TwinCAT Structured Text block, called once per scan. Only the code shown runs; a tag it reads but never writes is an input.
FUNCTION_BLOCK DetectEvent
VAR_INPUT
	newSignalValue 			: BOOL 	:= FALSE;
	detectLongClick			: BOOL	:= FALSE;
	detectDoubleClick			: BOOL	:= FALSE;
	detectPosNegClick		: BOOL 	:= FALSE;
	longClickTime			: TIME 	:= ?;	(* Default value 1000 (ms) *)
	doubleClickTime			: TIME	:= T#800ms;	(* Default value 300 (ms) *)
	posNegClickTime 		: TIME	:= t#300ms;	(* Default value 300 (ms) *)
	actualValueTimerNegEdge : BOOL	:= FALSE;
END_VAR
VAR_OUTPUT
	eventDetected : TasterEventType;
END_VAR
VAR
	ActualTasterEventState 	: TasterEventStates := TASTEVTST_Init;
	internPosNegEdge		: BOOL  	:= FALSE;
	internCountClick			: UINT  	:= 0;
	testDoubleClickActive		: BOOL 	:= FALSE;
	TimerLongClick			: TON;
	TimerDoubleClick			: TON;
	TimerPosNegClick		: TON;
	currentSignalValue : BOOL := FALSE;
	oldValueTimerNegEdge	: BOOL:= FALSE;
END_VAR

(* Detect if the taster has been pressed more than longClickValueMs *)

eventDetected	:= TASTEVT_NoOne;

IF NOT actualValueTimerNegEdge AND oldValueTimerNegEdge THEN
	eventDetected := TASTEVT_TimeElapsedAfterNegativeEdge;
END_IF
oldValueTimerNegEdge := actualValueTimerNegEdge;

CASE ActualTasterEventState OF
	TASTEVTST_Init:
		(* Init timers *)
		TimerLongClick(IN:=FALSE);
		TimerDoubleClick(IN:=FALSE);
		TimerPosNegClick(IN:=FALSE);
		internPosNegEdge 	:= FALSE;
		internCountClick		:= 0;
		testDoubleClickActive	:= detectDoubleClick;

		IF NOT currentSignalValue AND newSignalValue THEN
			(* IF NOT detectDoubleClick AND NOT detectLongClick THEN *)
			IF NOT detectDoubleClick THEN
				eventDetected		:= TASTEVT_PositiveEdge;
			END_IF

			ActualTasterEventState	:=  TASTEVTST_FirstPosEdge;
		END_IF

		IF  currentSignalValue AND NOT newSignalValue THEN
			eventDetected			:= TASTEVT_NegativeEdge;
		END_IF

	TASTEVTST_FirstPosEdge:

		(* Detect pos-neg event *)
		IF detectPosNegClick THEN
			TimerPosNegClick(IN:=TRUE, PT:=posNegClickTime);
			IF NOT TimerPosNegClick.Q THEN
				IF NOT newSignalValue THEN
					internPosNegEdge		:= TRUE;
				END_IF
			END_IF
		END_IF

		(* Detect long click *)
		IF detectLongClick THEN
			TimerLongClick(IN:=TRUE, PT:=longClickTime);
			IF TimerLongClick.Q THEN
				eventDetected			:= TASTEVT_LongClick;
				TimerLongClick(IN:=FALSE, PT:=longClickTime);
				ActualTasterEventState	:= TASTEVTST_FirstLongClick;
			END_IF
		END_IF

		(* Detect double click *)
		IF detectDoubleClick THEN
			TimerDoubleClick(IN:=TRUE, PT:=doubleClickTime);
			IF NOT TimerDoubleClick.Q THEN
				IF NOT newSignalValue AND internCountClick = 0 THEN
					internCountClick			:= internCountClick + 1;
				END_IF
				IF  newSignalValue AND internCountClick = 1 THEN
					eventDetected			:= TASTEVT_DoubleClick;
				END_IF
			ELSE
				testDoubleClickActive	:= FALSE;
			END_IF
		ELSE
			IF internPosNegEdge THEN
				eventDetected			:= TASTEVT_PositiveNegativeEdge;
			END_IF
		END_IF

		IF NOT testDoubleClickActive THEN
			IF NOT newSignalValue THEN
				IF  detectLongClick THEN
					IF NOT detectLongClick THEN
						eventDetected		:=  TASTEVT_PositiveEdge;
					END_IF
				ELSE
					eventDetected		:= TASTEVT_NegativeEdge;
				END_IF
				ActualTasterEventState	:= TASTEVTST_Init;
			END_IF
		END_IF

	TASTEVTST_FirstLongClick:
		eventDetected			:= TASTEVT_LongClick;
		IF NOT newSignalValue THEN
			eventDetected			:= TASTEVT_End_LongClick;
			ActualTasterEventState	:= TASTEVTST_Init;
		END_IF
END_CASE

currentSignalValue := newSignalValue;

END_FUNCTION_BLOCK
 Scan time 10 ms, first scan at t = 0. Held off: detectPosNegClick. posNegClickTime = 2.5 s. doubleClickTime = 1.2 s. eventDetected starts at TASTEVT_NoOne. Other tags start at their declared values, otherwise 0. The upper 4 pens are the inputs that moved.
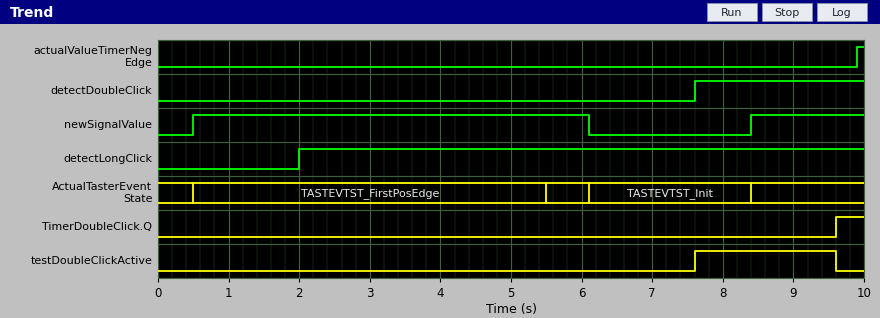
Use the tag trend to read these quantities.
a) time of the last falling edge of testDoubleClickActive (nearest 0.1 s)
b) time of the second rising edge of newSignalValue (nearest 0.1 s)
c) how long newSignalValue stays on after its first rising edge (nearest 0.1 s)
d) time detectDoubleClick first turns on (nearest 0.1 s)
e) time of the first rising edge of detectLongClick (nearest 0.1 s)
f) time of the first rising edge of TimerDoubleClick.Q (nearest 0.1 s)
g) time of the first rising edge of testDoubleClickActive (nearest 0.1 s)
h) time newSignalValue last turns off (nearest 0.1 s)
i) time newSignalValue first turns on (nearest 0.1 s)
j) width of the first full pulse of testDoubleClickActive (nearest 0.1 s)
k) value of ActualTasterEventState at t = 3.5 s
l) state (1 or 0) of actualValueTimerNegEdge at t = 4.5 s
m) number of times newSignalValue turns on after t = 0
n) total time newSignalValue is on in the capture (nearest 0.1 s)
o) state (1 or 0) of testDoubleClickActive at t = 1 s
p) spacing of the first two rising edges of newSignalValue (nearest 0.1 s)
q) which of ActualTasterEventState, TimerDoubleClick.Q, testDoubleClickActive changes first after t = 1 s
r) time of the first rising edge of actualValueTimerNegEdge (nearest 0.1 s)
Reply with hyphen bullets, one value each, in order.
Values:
- 9.6 s
- 8.4 s
- 5.6 s
- 7.6 s
- 2.0 s
- 9.6 s
- 7.6 s
- 6.1 s
- 0.5 s
- 2.0 s
- TASTEVTST_FirstPosEdge
- 0
- 2
- 7.2 s
- 0
- 7.9 s
- ActualTasterEventState
- 9.9 s
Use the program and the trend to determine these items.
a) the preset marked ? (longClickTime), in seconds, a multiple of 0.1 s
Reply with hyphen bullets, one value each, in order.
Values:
- 3.5 s
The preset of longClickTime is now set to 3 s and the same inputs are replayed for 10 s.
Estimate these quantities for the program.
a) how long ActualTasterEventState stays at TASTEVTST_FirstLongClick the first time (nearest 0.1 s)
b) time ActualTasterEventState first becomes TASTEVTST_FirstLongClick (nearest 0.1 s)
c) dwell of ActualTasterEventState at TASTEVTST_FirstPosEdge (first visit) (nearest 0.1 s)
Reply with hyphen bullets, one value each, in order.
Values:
- 1.1 s
- 5.0 s
- 4.5 s
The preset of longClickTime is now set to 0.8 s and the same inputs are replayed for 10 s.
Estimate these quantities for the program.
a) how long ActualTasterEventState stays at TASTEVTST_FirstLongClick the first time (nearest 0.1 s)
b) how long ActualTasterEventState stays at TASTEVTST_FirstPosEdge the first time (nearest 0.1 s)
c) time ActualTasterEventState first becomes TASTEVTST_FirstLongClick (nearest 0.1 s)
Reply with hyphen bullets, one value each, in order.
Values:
- 3.3 s
- 2.3 s
- 2.8 s
